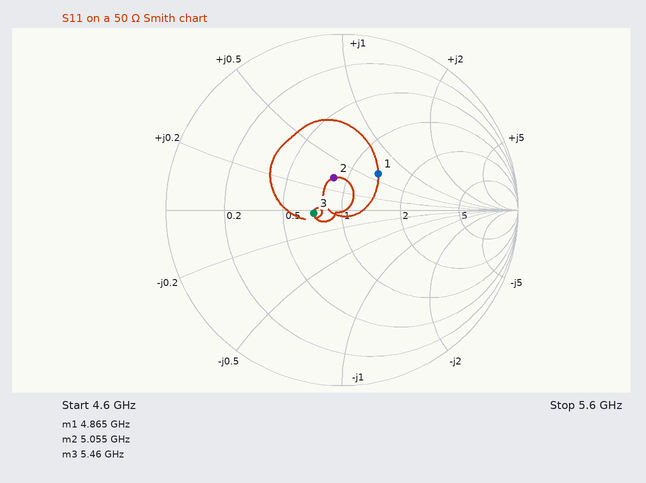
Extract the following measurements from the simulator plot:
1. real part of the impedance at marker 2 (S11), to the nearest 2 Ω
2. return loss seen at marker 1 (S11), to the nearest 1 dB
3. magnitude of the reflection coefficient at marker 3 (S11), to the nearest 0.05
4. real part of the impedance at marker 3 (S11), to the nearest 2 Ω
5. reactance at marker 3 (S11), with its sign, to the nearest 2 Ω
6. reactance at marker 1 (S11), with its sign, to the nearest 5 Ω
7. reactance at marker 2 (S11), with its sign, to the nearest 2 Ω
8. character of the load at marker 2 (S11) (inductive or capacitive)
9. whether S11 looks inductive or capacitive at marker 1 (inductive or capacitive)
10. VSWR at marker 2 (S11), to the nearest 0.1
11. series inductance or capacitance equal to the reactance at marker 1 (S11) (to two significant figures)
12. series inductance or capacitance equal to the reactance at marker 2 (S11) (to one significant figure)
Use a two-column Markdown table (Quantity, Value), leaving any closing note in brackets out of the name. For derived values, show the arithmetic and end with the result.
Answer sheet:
| Quantity | Value |
|---|---|
| real part of the impedance at marker 2 (S11), to the nearest 2 Ω | 42 Ω |
| return loss seen at marker 1 (S11), to the nearest 1 dB | 11 dB |
| magnitude of the reflection coefficient at marker 3 (S11), to the nearest 0.05 | 0.15 |
| real part of the impedance at marker 3 (S11), to the nearest 2 Ω | 36 Ω |
| reactance at marker 3 (S11), with its sign, to the nearest 2 Ω | -2 Ω |
| reactance at marker 1 (S11), with its sign, to the nearest 5 Ω | +30 Ω |
| reactance at marker 2 (S11), with its sign, to the nearest 2 Ω | +16 Ω |
| character of the load at marker 2 (S11) | inductive |
| whether S11 looks inductive or capacitive at marker 1 | inductive |
| VSWR at marker 2 (S11), to the nearest 0.1 | 1.5 |
| series inductance or capacitance equal to the reactance at marker 1 (S11) | L = 30 Ω/(2π × 4.865 GHz) ≈ 1.0 nH |
| series inductance or capacitance equal to the reactance at marker 2 (S11) | L = 16 Ω/(2π × 5.055 GHz) ≈ 504 pH, so 500 pH to one significant figure |
